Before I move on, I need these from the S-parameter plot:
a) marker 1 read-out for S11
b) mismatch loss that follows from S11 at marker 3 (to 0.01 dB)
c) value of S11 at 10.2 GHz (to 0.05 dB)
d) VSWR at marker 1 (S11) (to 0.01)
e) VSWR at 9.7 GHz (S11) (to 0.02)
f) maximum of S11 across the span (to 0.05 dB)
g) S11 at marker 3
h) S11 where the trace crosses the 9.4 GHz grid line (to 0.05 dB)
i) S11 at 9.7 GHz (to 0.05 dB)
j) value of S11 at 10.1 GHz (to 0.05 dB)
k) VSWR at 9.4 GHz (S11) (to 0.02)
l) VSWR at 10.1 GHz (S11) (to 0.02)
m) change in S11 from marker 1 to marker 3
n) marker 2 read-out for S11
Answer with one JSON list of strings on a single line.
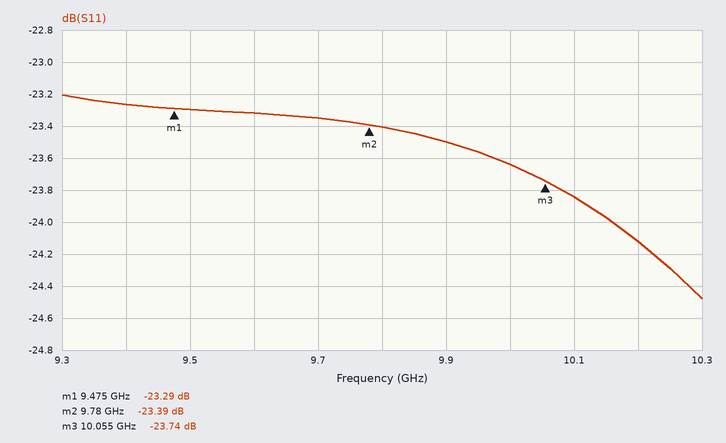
["-23.29 dB", "0.02 dB", "-24.10 dB", "1.15", "1.14", "-23.20 dB", "-23.74 dB", "-23.25 dB", "-23.35 dB", "-23.85 dB", "1.14", "1.14", "-0.45 dB", "-23.39 dB"]
